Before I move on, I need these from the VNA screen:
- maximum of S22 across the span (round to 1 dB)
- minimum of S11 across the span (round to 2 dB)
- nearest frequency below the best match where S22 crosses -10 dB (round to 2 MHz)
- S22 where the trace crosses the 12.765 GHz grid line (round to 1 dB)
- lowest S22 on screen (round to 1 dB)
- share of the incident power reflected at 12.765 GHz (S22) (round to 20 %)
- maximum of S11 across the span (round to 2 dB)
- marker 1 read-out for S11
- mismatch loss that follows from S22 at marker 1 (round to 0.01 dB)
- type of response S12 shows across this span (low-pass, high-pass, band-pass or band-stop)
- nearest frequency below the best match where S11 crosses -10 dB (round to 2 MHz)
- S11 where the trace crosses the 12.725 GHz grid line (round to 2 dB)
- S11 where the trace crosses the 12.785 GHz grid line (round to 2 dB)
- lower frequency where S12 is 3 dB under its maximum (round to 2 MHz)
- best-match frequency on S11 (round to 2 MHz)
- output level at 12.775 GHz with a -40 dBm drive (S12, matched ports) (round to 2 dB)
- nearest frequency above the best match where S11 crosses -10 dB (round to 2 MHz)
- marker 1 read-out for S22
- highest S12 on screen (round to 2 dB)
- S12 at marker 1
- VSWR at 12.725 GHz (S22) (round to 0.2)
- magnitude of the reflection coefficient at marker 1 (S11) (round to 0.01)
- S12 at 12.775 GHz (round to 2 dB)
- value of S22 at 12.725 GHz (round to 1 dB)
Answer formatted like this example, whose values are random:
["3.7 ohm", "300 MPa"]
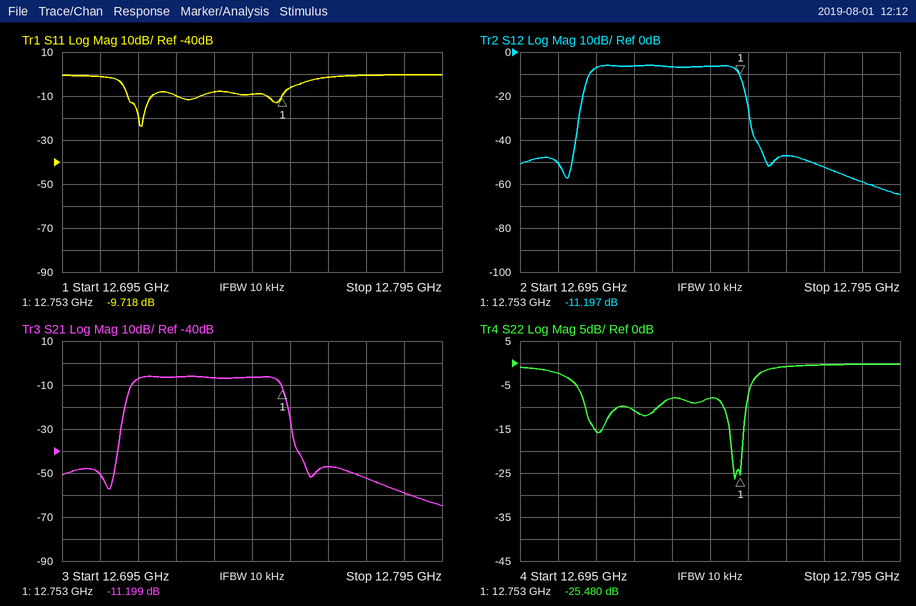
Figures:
["0 dB", "-24 dB", "12.748 GHz", "-1 dB", "-26 dB", "80 %", "0 dB", "-9.718 dB", "0.01 dB", "band-pass", "12.712 GHz", "-10 dB", "0 dB", "12.714 GHz", "12.716 GHz", "-92 dBm", "12.718 GHz", "-25.480 dB", "-6 dB", "-11.197 dB", "1.8", "0.33", "-52 dB", "-11 dB"]
